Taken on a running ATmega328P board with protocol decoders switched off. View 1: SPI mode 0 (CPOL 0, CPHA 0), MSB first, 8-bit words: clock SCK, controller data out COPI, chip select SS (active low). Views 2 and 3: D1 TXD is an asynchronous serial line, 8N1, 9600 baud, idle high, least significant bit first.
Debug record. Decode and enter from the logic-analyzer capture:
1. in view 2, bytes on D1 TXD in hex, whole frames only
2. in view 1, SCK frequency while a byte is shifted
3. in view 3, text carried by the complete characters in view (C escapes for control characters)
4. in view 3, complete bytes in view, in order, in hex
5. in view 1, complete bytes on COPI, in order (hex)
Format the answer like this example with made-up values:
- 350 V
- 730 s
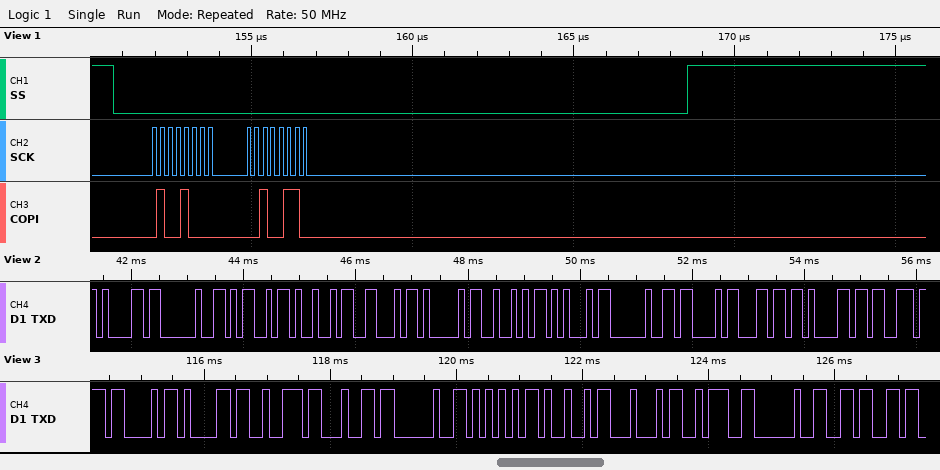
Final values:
- 61 20 4D 49 46 41 52 45 20 43 6C 61 73
- 4 MHz
- "Card UID: 6"
- 43 61 72 64 20 55 49 44 3A 20 36
- 48 26
